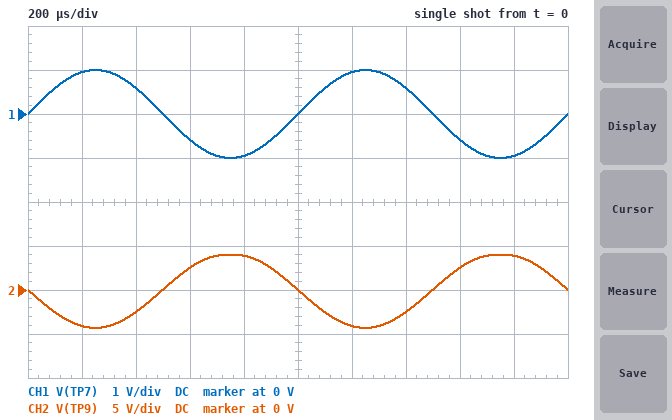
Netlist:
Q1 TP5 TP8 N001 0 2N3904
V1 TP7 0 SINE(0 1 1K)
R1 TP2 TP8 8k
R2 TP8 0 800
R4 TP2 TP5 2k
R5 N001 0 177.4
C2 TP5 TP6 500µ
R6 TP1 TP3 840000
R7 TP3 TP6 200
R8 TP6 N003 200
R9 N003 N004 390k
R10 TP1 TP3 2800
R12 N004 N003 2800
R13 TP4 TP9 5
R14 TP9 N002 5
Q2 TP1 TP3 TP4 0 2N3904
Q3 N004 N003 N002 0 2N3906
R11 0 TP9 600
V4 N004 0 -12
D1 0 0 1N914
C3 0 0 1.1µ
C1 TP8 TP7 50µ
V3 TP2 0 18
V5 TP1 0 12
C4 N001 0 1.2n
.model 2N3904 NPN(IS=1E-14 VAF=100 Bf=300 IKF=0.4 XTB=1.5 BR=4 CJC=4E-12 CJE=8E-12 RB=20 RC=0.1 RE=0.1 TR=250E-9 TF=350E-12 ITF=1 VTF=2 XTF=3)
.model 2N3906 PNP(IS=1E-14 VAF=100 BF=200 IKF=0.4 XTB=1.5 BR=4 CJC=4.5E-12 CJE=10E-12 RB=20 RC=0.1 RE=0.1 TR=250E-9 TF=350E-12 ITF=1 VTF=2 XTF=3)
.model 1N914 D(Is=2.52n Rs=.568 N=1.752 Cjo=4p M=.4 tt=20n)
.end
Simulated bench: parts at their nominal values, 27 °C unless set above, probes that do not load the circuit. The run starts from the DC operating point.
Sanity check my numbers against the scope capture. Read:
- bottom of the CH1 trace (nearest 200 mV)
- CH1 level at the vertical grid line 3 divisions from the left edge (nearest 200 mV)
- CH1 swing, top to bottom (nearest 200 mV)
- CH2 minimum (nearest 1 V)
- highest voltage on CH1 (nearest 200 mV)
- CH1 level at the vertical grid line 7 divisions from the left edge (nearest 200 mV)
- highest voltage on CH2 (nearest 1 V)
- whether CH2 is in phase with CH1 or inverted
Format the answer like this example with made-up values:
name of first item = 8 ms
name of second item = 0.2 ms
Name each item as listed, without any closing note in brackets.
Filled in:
bottom of the CH1 trace = -1.0 V
CH1 level at the vertical grid line 3 divisions from the left edge = -600 mV
CH1 swing, top to bottom = 2.0 V
CH2 minimum = -4 V
highest voltage on CH1 = 1.0 V
CH1 level at the vertical grid line 7 divisions from the left edge = 600 mV
highest voltage on CH2 = 4 V
whether CH2 is in phase with CH1 or inverted = inverted
